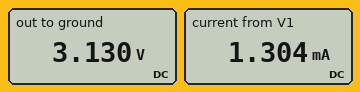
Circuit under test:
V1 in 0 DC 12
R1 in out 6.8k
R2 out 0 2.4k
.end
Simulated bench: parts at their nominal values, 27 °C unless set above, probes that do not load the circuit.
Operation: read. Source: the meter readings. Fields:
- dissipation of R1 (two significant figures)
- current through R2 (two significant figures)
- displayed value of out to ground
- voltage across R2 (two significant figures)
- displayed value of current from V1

12 mW
1.3 mA
3.130 V
3.1 V
1.304 mA
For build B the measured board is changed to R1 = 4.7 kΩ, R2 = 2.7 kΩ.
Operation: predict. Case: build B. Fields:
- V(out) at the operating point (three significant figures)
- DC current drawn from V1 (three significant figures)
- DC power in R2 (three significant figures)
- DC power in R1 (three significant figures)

4.38 V
1.62 mA
7.10 mW
12.4 mW
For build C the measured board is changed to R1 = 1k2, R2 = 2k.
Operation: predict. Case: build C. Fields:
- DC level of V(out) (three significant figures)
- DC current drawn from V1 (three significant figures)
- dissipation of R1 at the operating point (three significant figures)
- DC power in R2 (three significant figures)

7.50 V
3.75 mA
16.9 mW
28.1 mW
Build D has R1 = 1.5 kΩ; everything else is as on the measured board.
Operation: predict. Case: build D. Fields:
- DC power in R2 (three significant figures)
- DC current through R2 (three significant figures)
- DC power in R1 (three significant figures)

22.7 mW
3.08 mA
14.2 mW
